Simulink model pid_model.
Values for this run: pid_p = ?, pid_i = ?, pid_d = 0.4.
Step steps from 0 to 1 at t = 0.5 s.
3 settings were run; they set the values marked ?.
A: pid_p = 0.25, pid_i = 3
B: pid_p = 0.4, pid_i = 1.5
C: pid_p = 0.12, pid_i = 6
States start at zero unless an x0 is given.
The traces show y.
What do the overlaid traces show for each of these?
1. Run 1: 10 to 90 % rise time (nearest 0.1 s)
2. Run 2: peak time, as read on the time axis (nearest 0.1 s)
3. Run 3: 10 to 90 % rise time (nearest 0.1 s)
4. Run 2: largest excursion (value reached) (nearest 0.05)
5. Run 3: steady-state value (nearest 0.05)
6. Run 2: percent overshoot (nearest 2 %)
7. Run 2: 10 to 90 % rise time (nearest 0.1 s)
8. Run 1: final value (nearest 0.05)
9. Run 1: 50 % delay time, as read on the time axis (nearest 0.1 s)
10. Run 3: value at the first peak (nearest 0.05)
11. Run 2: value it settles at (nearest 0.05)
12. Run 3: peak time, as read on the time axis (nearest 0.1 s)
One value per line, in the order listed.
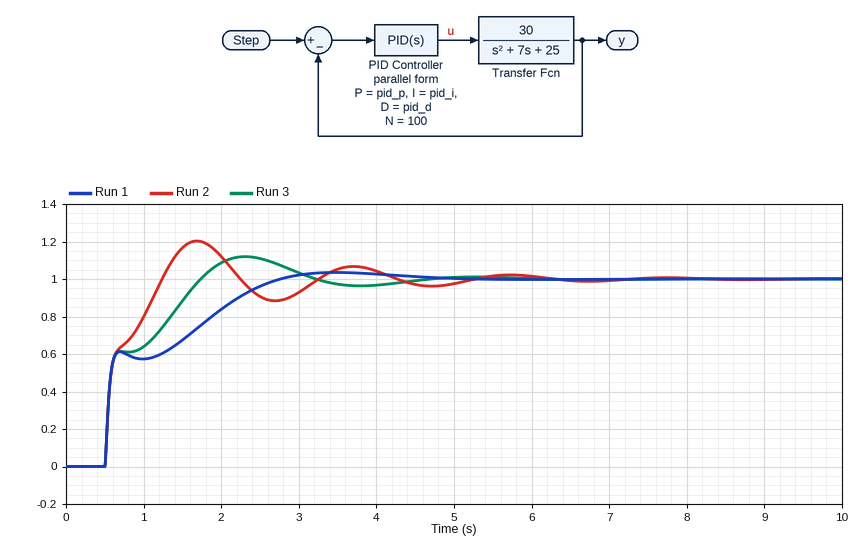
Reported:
1.7 s
1.7 s
1.0 s
1.20
1.00
20 %
0.6 s
1.00
0.6 s
1.10
1.00
2.3 s
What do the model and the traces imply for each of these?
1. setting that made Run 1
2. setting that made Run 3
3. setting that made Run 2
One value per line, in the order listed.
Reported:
B
A
C
